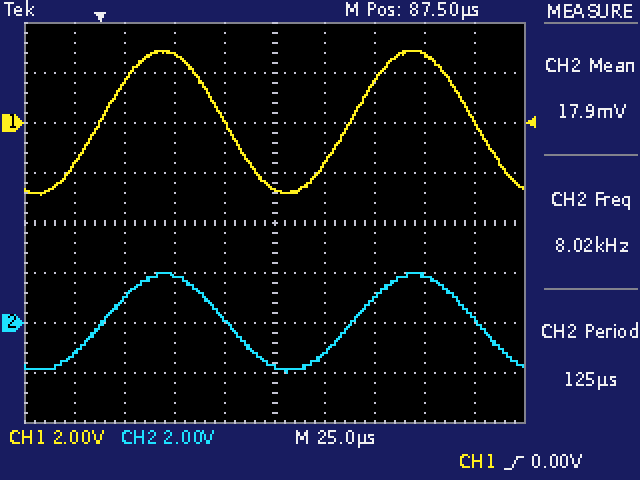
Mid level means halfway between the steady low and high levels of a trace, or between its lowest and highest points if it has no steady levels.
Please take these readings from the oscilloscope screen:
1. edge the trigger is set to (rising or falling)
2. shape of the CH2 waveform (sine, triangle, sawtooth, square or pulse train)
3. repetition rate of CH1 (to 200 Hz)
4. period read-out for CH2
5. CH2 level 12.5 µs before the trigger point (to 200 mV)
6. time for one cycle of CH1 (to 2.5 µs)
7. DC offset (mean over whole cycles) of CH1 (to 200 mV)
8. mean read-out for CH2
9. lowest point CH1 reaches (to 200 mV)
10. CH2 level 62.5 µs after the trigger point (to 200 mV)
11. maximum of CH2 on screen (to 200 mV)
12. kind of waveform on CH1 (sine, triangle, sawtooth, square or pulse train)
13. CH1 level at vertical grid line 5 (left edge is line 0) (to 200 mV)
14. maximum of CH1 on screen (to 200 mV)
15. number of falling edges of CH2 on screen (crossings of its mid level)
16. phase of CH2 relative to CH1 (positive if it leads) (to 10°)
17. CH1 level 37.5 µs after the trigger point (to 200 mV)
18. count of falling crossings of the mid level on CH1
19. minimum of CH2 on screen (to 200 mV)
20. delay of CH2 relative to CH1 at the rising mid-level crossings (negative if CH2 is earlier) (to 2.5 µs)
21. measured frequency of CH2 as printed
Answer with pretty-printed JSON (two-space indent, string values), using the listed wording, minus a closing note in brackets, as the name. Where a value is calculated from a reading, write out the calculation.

{
  "edge the trigger is set to": "rising",
  "shape of the CH2 waveform": "sine",
  "repetition rate of CH1": "1 / 125.0 µs ≈ 8.0 kHz",
  "period read-out for CH2": "125 µs",
  "CH2 level 12.5 µs before the trigger point": "-1.2 V",
  "time for one cycle of CH1": "125.0 µs",
  "DC offset (mean over whole cycles) of CH1": "(2.8 V + (-2.8 V)) / 2 ≈ 0.0 V",
  "mean read-out for CH2": "17.9 mV",
  "lowest point CH1 reaches": "-2.8 V",
  "CH2 level 62.5 µs after the trigger point": "200 mV",
  "maximum of CH2 on screen": "2.0 V",
  "kind of waveform on CH1": "sine",
  "CH1 level at vertical grid line 5 (left edge is line 0)": "-2.6 V",
  "maximum of CH1 on screen": "2.8 V",
  "number of falling edges of CH2 on screen": "2",
  "phase of CH2 relative to CH1 (positive if it leads)": "−360° × (0.0 µs) / 125.0 µs ≈ 0°",
  "CH1 level 37.5 µs after the trigger point": "2.8 V",
  "count of falling crossings of the mid level on CH1": "2",
  "minimum of CH2 on screen": "-2.0 V",
  "delay of CH2 relative to CH1 at the rising mid-level crossings (negative if CH2 is earlier)": "0.0 µs",
  "measured frequency of CH2 as printed": "8.02 kHz"
}
